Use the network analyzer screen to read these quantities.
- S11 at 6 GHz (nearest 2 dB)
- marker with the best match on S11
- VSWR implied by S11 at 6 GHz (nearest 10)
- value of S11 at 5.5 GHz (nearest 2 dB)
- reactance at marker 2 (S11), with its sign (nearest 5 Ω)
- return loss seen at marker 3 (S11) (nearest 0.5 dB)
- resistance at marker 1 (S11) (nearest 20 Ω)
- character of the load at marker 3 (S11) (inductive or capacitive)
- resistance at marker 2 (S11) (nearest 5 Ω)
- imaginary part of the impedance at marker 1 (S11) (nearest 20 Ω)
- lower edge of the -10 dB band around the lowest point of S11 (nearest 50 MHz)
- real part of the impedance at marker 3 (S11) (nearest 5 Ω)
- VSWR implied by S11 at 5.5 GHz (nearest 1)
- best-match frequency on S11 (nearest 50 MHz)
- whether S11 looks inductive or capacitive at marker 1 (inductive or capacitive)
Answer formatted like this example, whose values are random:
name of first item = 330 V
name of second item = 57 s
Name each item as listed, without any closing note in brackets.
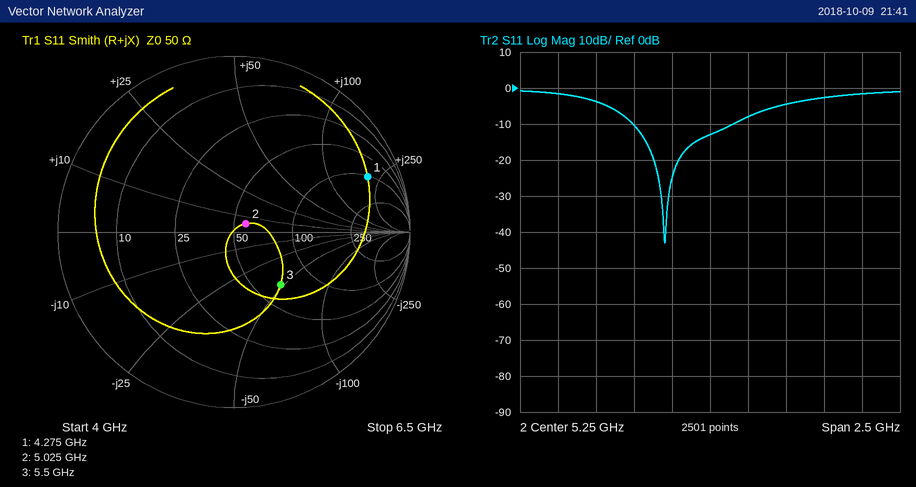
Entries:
S11 at 6 GHz = -2 dB
marker with the best match on S11 = marker 2
VSWR implied by S11 at 6 GHz = 10
value of S11 at 5.5 GHz = -8 dB
reactance at marker 2 (S11), with its sign = +5 Ω
return loss seen at marker 3 (S11) = 8.0 dB
resistance at marker 1 (S11) = 100 Ω
character of the load at marker 3 (S11) = capacitive
resistance at marker 2 (S11) = 55 Ω
imaginary part of the impedance at marker 1 (S11) = +200 Ω
lower edge of the -10 dB band around the lowest point of S11 = 4.75 GHz
real part of the impedance at marker 3 (S11) = 65 Ω
VSWR implied by S11 at 5.5 GHz = 2
best-match frequency on S11 = 4.95 GHz
whether S11 looks inductive or capacitive at marker 1 = inductive
